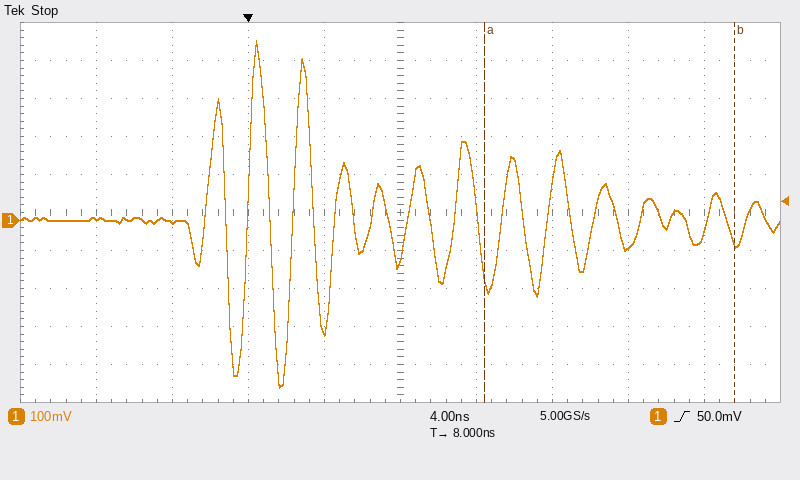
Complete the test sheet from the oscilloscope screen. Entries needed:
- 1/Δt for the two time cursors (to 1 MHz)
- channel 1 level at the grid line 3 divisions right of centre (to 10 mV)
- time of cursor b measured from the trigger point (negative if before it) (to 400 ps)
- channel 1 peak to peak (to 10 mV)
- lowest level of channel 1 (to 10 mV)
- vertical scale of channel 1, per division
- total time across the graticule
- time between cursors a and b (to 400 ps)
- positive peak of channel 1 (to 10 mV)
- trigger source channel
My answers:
76 MHz
-70 mV
+25.6 ns
910 mV
-440 mV
100 mV
40 ns
13.2 ns
470 mV
channel 1
